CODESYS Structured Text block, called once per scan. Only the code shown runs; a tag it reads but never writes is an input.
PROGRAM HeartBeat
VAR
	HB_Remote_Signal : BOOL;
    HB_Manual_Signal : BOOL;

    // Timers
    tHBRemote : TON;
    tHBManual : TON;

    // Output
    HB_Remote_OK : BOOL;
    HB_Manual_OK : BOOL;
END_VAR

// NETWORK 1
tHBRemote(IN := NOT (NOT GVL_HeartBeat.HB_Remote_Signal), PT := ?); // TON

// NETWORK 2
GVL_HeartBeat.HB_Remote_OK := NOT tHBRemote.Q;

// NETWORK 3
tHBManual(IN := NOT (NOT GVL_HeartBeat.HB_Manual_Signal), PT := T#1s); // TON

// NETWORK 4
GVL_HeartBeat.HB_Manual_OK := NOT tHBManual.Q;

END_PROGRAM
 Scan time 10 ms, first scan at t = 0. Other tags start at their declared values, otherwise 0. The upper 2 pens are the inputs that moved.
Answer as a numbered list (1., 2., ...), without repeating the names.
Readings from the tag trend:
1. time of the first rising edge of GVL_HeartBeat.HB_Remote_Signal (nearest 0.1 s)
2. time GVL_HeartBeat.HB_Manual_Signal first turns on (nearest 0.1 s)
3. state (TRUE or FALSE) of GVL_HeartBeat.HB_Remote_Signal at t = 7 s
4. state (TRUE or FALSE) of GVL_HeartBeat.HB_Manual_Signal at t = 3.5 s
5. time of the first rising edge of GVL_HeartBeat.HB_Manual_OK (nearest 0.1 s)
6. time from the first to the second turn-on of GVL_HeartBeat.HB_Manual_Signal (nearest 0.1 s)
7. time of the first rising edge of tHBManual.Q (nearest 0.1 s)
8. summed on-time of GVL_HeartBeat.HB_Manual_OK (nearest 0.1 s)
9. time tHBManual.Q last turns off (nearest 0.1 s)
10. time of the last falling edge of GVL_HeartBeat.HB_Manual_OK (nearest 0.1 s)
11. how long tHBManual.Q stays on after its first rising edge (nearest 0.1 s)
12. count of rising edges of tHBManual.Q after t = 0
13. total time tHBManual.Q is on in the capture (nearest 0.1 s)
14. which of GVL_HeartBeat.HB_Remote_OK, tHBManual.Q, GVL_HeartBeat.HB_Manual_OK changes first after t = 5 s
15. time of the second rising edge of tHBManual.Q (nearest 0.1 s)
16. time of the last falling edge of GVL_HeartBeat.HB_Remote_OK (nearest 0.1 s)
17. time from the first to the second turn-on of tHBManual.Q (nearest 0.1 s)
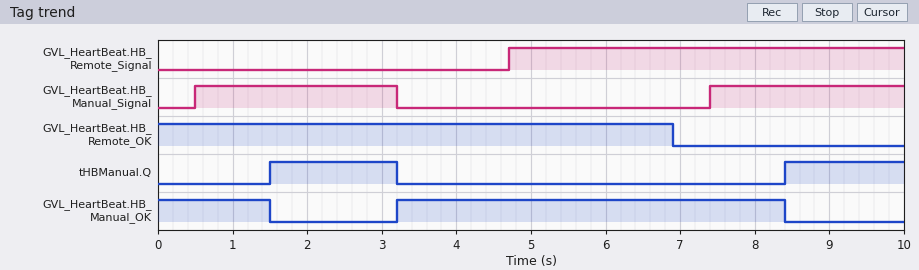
1. 4.7 s
2. 0.5 s
3. TRUE
4. FALSE
5. 3.2 s
6. 6.9 s
7. 1.5 s
8. 6.7 s
9. 3.2 s
10. 8.4 s
11. 1.7 s
12. 2
13. 3.3 s
14. GVL_HeartBeat.HB_Remote_OK
15. 8.4 s
16. 6.9 s
17. 6.9 s
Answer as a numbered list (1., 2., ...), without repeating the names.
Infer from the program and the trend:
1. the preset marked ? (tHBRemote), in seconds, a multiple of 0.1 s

1. 2.2 s
